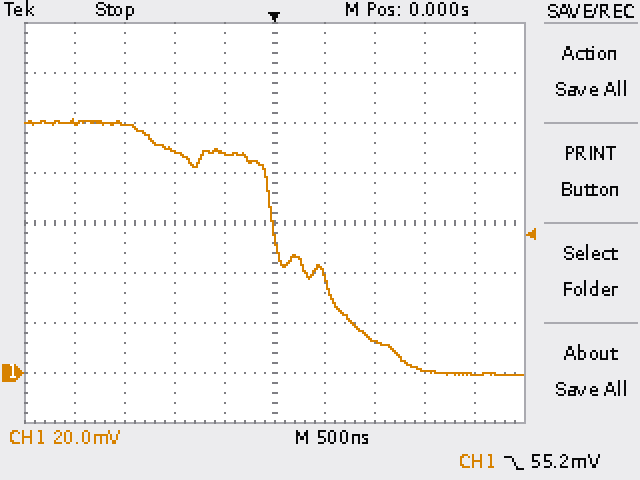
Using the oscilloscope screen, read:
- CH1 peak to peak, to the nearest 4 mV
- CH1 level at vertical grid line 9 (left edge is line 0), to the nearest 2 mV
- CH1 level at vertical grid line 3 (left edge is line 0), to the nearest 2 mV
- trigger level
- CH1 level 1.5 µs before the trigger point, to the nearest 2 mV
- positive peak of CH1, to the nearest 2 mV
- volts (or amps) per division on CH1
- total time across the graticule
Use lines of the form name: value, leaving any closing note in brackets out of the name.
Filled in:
CH1 peak to peak, to the nearest 4 mV: 104 mV
CH1 level at vertical grid line 9 (left edge is line 0), to the nearest 2 mV: 0 mV
CH1 level at vertical grid line 3 (left edge is line 0), to the nearest 2 mV: 88 mV
trigger level: 55.2 mV
CH1 level 1.5 µs before the trigger point, to the nearest 2 mV: 100 mV
positive peak of CH1, to the nearest 2 mV: 102 mV
volts (or amps) per division on CH1: 20 mV
total time across the graticule: 5 µs
